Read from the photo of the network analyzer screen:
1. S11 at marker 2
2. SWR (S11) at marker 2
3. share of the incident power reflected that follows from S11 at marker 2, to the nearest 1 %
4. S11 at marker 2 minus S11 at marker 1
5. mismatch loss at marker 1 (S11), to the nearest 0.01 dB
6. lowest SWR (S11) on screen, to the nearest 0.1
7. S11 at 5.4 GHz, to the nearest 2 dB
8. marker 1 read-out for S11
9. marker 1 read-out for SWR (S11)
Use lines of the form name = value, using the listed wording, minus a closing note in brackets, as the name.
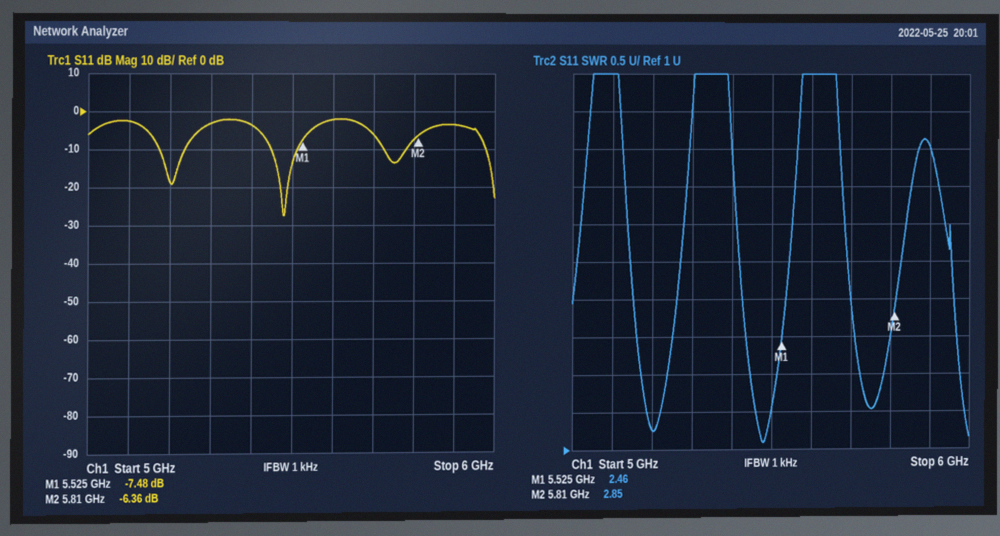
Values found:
S11 at marker 2 = -6.36 dB
SWR (S11) at marker 2 = 2.85
share of the incident power reflected that follows from S11 at marker 2, to the nearest 1 % = 23 %
S11 at marker 2 minus S11 at marker 1 = 1.12 dB
mismatch loss at marker 1 (S11), to the nearest 0.01 dB = 0.85 dB
lowest SWR (S11) on screen, to the nearest 0.1 = 1.1
S11 at 5.4 GHz, to the nearest 2 dB = -4 dB
marker 1 read-out for S11 = -7.48 dB
marker 1 read-out for SWR = 2.46
